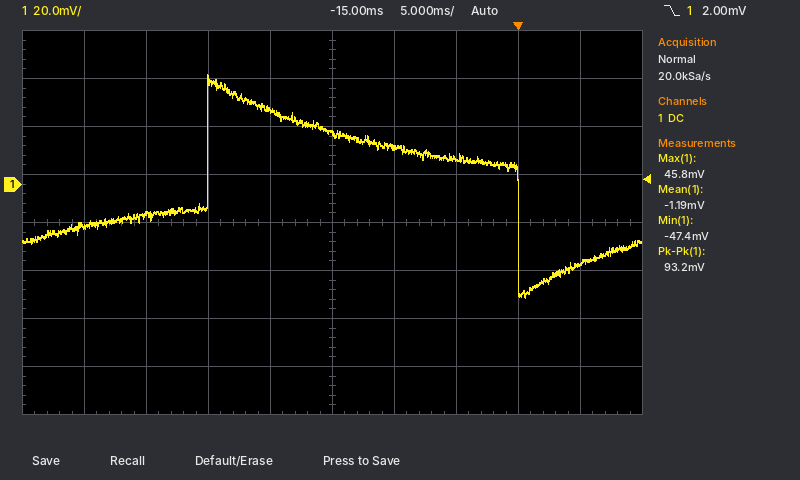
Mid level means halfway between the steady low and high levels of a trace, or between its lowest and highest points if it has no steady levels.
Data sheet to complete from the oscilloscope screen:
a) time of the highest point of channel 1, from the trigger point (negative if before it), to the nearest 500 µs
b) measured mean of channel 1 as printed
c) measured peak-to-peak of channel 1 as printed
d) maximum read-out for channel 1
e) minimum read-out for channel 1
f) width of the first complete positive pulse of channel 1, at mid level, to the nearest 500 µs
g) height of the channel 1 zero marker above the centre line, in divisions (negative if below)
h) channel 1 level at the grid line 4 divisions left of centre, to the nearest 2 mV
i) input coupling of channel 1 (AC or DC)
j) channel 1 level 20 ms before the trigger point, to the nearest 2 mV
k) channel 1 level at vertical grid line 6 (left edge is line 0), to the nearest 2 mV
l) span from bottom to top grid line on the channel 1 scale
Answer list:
-25.0 ms
-1.19 mV
93.2 mV
45.8 mV
-47.4 mV
25.0 ms
+0.8 div
-18 mV
DC
32 mV
16 mV
160 mV
